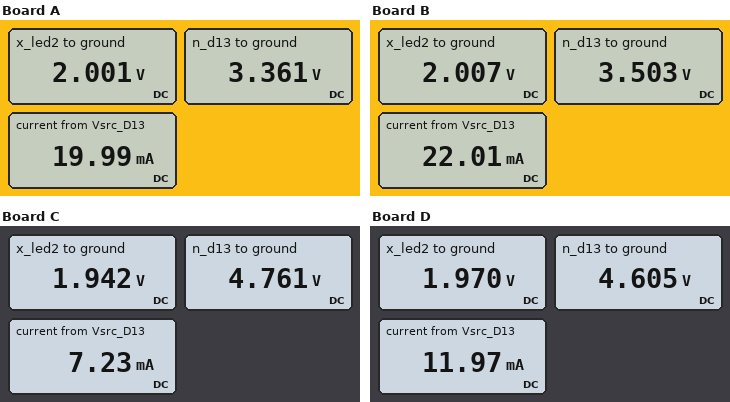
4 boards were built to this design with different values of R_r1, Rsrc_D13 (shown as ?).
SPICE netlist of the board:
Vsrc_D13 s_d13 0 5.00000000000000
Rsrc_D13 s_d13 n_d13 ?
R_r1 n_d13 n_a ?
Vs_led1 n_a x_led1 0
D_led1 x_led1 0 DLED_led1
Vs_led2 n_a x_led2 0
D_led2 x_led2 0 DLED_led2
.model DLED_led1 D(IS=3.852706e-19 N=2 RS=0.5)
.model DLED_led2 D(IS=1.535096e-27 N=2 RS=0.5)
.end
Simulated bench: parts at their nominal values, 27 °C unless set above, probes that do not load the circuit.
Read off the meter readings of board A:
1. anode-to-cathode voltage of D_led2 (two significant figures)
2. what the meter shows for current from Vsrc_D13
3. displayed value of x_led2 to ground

2.0 V
19.99 mA
2.001 V
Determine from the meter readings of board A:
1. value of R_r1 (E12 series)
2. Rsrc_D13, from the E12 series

68 Ω
82 Ω
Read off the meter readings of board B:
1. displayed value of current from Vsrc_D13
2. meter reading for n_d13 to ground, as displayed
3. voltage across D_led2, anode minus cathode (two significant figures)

22.01 mA
3.503 V
2.0 V
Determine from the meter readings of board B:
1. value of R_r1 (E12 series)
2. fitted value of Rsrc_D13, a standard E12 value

68 Ω
68 Ω
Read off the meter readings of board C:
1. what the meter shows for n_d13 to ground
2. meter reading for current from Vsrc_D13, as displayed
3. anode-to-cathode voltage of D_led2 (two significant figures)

4.761 V
7.23 mA
1.9 V
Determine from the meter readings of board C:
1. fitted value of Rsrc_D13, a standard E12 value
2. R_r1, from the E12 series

33 Ω
390 Ω
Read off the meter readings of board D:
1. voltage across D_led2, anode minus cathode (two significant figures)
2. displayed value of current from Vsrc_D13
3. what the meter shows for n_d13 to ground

2.0 V
11.97 mA
4.605 V
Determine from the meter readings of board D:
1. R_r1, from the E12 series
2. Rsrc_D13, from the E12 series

220 Ω
33 Ω
